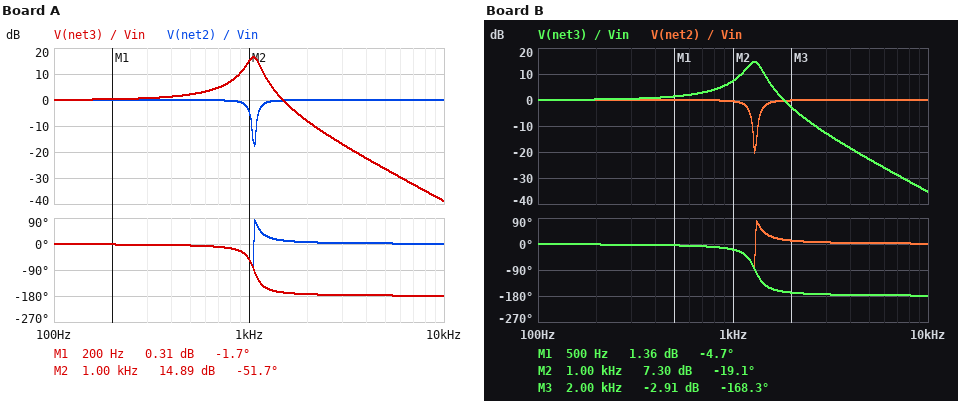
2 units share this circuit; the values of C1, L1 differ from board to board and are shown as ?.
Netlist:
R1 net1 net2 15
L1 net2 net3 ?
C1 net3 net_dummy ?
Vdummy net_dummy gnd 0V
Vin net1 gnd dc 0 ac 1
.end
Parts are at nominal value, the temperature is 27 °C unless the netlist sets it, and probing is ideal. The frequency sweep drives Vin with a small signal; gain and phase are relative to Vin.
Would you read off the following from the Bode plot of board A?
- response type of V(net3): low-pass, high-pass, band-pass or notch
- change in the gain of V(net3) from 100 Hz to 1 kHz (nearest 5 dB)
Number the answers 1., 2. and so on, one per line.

1. low-pass
2. 15 dB
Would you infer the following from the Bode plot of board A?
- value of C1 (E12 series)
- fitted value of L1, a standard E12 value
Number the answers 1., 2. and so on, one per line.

1. 1.5 µF
2. 15 mH
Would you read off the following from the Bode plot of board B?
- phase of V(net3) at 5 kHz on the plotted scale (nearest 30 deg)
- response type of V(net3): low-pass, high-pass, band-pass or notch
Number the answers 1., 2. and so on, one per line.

1. -180 deg
2. low-pass
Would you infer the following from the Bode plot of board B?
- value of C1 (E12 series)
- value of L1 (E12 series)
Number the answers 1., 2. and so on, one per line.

1. 1.5 µF
2. 10 mH
